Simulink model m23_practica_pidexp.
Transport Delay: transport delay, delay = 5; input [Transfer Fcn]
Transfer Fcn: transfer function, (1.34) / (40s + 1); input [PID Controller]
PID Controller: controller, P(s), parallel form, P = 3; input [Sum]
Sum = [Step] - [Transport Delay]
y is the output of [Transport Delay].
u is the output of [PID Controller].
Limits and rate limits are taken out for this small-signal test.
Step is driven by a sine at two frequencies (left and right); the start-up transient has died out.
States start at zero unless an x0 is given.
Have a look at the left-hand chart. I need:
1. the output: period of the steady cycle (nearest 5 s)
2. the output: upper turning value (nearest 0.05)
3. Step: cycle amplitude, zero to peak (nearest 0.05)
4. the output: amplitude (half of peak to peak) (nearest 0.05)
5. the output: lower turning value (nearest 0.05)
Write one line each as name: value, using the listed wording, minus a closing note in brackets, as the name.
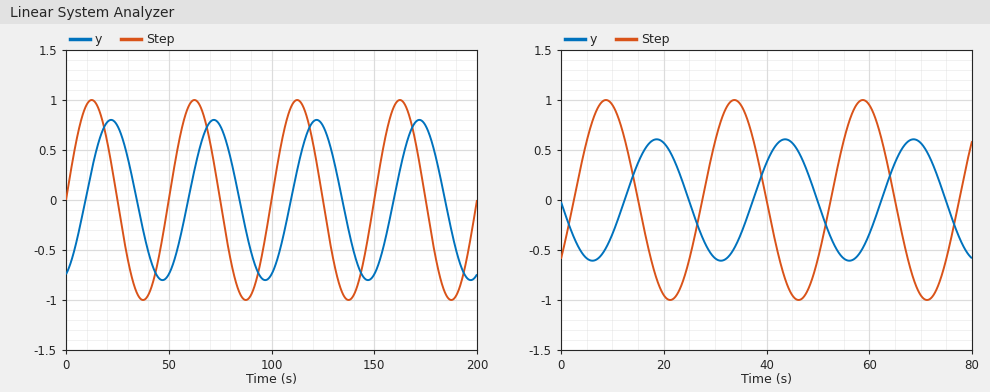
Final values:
the output: period of the steady cycle: 50 s
the output: upper turning value: 0.80
Step: cycle amplitude, zero to peak: 1.00
the output: amplitude (half of peak to peak): 0.80
the output: lower turning value: -0.80
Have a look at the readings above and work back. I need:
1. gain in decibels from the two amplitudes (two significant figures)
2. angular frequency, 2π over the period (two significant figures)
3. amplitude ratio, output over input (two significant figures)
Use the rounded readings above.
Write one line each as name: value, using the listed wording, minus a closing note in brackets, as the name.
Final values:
gain in decibels from the two amplitudes: -1.9 dB
angular frequency, 2π over the period: 0.13 rad/s
amplitude ratio, output over input: 0.80
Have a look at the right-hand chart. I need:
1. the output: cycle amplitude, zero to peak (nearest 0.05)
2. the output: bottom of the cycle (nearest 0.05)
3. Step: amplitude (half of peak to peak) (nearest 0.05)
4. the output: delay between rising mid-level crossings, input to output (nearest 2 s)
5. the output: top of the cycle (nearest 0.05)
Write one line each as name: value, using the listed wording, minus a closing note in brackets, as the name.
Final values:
the output: cycle amplitude, zero to peak: 0.60
the output: bottom of the cycle: -0.60
Step: amplitude (half of peak to peak): 1.00
the output: delay between rising mid-level crossings, input to output: 10 s
the output: top of the cycle: 0.60
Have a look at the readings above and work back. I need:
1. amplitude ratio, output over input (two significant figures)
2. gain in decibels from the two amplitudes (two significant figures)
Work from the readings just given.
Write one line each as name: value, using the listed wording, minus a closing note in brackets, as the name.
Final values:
amplitude ratio, output over input: 0.60
gain in decibels from the two amplitudes: -4.4 dB
